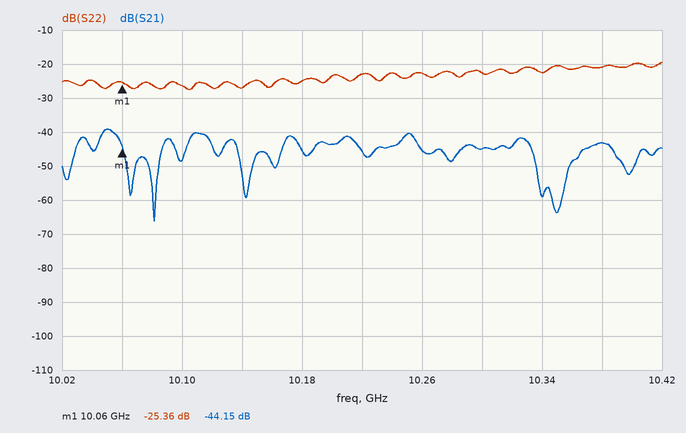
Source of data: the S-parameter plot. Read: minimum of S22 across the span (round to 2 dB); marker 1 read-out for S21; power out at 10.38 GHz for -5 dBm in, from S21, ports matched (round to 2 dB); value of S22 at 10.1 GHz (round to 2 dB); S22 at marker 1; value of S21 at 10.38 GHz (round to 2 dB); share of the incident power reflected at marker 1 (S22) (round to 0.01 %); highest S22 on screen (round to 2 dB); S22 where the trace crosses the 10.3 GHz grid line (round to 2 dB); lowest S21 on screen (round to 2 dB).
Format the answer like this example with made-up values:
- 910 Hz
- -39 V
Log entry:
- -28 dB
- -44.15 dB
- -48 dBm
- -26 dB
- -25.36 dB
- -44 dB
- 0.29 %
- -20 dB
- -22 dB
- -66 dB
